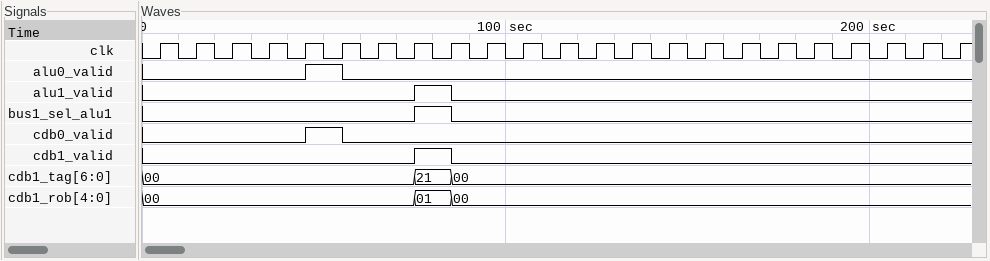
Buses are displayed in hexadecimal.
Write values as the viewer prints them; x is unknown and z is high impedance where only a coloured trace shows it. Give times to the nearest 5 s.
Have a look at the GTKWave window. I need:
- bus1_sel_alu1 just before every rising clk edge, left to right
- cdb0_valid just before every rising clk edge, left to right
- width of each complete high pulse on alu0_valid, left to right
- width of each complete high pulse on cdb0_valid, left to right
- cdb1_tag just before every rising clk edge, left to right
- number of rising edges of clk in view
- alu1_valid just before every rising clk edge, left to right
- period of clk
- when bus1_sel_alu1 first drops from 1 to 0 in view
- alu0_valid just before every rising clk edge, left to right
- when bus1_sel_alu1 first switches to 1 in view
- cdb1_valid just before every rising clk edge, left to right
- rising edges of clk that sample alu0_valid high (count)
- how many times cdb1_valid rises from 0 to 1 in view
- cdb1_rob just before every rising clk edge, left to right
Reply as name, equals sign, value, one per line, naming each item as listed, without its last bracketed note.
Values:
bus1_sel_alu1 just before every rising clk edge, left to right = 0 0 0 0 0 0 0 0 1 0 0 0 0 0 0 0 0 0 0 0 0 0 0
cdb0_valid just before every rising clk edge, left to right = 0 0 0 0 0 1 0 0 0 0 0 0 0 0 0 0 0 0 0 0 0 0 0
width of each complete high pulse on alu0_valid, left to right = 10 s
width of each complete high pulse on cdb0_valid, left to right = 10 s
cdb1_tag just before every rising clk edge, left to right = 00, 00, 00, 00, 00, 00, 00, 00, 21, 00, 00, 00, 00, 00, 00, 00, 00, 00, 00, 00, 00, 00, 00
number of rising edges of clk in view = 23
alu1_valid just before every rising clk edge, left to right = 0 0 0 0 0 0 0 0 1 0 0 0 0 0 0 0 0 0 0 0 0 0 0
period of clk = 10 s
when bus1_sel_alu1 first drops from 1 to 0 in view = 85 s
alu0_valid just before every rising clk edge, left to right = 0 0 0 0 0 1 0 0 0 0 0 0 0 0 0 0 0 0 0 0 0 0 0
when bus1_sel_alu1 first switches to 1 in view = 75 s
cdb1_valid just before every rising clk edge, left to right = 0 0 0 0 0 0 0 0 1 0 0 0 0 0 0 0 0 0 0 0 0 0 0
rising edges of clk that sample alu0_valid high = 1
how many times cdb1_valid rises from 0 to 1 in view = 1
cdb1_rob just before every rising clk edge, left to right = 00, 00, 00, 00, 00, 00, 00, 00, 01, 00, 00, 00, 00, 00, 00, 00, 00, 00, 00, 00, 00, 00, 00
